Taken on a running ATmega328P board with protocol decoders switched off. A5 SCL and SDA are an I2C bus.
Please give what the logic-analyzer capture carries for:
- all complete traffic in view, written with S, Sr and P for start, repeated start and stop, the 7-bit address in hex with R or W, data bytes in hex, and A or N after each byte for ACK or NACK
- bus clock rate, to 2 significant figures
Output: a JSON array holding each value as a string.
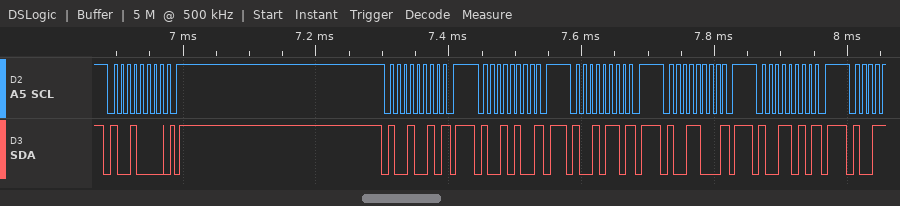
["S 48W A P S 49W N P S 4AW N P S 4BW N P S 4CW N P S 4DW N P", "100 kHz"]
